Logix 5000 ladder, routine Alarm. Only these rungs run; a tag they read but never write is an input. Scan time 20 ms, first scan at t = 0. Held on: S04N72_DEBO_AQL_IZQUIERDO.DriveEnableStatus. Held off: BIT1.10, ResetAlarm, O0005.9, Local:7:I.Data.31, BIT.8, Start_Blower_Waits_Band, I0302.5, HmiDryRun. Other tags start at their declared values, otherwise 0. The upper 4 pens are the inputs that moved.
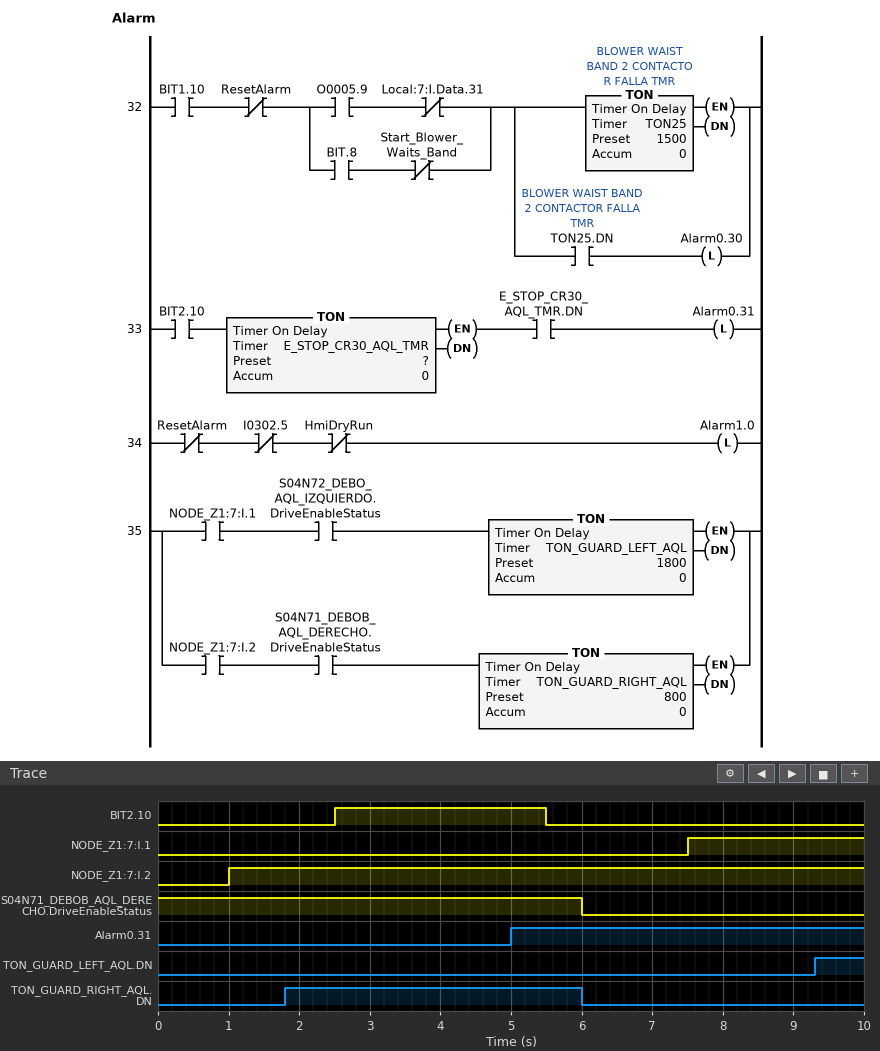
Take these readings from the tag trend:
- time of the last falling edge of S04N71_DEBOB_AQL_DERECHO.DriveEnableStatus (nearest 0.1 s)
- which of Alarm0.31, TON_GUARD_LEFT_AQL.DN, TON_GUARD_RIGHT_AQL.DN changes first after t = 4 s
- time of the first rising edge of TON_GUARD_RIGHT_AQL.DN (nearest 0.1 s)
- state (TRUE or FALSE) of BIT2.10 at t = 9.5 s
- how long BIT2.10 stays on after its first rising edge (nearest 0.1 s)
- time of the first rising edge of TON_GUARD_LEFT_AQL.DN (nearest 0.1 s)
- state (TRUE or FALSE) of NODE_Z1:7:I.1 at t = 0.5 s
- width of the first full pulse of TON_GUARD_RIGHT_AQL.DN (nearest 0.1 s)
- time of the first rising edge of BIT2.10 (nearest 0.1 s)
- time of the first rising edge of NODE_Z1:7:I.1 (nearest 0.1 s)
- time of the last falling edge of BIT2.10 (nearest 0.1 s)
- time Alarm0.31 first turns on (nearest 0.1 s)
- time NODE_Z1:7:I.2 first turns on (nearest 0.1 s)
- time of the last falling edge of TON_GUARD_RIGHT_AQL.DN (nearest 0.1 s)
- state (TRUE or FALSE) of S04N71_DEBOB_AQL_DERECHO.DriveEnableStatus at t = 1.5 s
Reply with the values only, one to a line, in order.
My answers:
6.0 s
Alarm0.31
1.8 s
FALSE
3.0 s
9.3 s
FALSE
4.2 s
2.5 s
7.5 s
5.5 s
5.0 s
1.0 s
6.0 s
TRUE
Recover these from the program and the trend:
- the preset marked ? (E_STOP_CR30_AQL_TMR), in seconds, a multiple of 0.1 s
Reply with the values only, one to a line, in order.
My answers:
2.5 s
